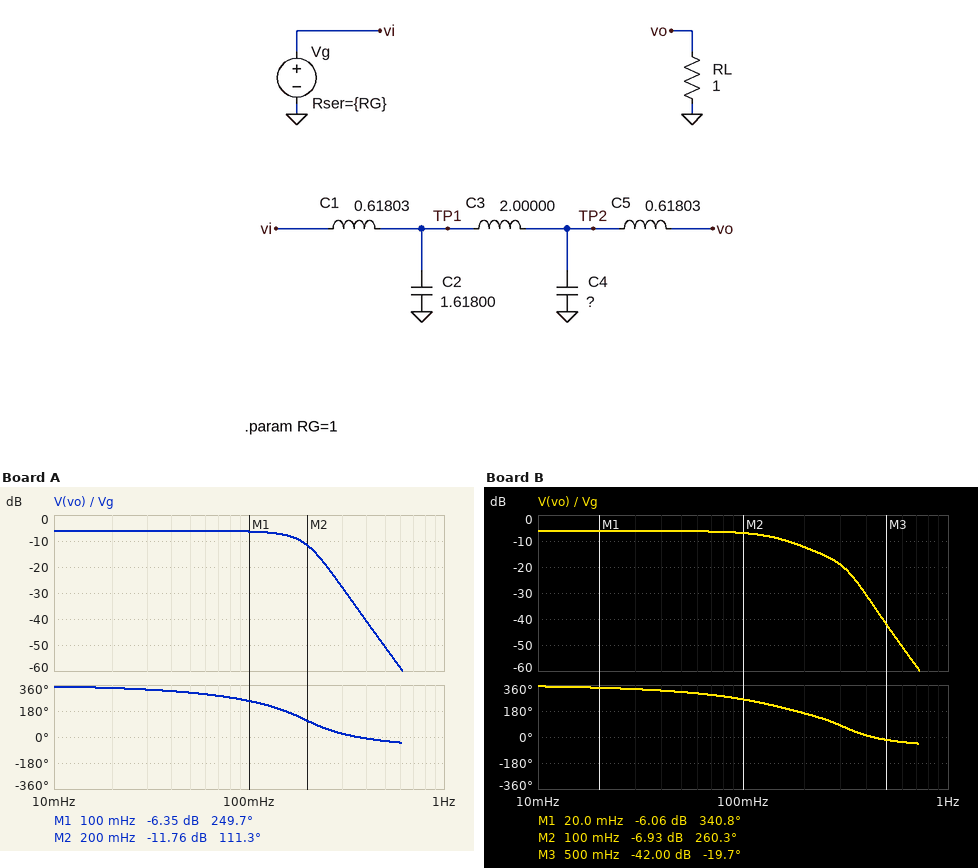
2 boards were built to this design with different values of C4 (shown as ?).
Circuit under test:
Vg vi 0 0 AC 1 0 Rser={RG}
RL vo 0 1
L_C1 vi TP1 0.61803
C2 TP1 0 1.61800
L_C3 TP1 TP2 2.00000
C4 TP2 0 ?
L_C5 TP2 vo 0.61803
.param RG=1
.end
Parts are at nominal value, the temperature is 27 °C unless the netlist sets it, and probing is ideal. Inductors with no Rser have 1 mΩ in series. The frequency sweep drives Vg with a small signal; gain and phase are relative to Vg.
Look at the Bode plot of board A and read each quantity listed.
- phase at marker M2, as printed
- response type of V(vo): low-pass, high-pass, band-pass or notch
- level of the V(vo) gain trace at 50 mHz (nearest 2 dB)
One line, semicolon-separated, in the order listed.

111.3 deg; low-pass; -6 dB
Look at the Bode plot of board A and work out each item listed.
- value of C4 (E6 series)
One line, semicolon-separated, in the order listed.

1 F
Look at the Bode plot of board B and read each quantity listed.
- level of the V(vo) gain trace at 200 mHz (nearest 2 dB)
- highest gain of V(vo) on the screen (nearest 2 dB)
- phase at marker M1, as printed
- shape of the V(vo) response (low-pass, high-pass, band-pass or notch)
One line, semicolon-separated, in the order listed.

-12 dB; -6 dB; 340.8 deg; low-pass
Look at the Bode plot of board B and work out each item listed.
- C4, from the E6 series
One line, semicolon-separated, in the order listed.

470 mF
